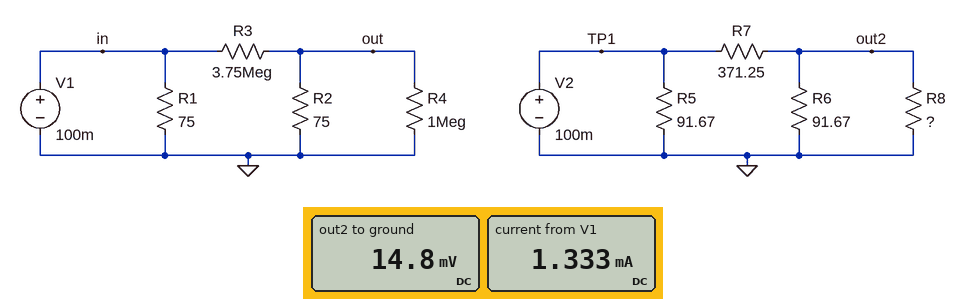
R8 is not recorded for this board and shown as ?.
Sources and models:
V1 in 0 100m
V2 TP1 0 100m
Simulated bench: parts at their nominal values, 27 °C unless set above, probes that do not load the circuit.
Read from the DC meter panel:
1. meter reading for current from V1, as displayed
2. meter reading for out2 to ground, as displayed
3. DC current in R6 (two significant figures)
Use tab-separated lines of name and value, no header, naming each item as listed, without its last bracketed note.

meter reading for current from V1, as displayed	1.333 mA
meter reading for out2 to ground, as displayed	14.8 mV
DC current in R6	160 µA
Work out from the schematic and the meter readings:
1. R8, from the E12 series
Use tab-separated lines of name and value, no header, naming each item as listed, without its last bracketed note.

R8, from the E12 series	220 Ω
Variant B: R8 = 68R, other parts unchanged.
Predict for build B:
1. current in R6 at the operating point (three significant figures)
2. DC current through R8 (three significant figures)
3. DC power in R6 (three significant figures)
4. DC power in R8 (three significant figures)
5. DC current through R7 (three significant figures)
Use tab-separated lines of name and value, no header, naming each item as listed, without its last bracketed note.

current in R6 at the operating point	104 µA
DC current through R8	140 µA
DC power in R6	988 nW
DC power in R8	1.33 µW
DC current through R7	244 µA
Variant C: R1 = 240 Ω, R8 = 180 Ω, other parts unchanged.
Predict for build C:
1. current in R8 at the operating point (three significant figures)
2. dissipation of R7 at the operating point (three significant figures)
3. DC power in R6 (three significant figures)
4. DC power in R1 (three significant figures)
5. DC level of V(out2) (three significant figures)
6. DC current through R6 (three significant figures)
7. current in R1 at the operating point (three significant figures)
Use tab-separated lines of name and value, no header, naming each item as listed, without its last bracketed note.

current in R8 at the operating point	78.1 µA
dissipation of R7 at the operating point	19.9 µW
DC power in R6	2.16 µW
DC power in R1	41.7 µW
DC level of V(out2)	14.1 mV
DC current through R6	153 µA
current in R1 at the operating point	417 µA
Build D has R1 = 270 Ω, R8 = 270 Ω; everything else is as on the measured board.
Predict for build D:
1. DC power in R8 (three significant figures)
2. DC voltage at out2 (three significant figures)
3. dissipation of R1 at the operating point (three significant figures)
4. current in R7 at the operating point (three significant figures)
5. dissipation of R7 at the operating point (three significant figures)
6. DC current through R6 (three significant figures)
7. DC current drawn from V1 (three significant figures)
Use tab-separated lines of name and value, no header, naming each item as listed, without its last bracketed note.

DC power in R8	897 nW
DC voltage at out2	15.6 mV
dissipation of R1 at the operating point	37.0 µW
current in R7 at the operating point	227 µA
dissipation of R7 at the operating point	19.2 µW
DC current through R6	170 µA
DC current drawn from V1	370 µA
